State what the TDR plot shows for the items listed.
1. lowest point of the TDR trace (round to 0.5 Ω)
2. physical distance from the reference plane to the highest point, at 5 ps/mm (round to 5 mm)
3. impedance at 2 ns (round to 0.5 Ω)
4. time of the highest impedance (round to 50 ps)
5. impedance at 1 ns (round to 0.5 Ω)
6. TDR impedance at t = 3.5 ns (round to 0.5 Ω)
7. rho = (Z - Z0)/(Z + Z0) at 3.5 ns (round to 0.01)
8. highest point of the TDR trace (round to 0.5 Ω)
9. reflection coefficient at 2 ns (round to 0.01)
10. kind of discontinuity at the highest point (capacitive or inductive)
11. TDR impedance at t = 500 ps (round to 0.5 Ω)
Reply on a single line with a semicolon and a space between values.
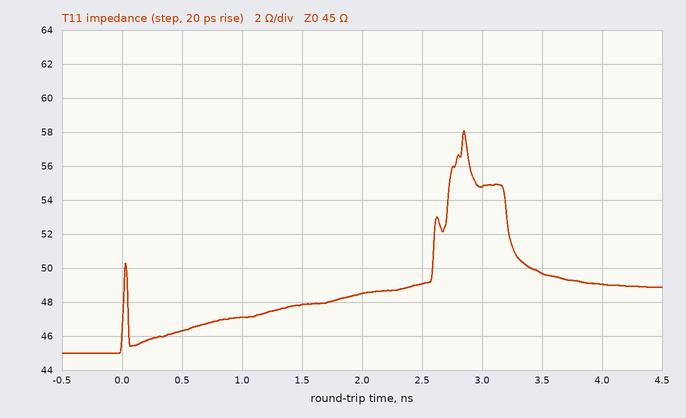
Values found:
45.0 Ω; 285 mm; 48.5 Ω; 2.85 ns; 47.0 Ω; 49.5 Ω; +0.05; 58.0 Ω; +0.04; inductive; 46.5 Ω
